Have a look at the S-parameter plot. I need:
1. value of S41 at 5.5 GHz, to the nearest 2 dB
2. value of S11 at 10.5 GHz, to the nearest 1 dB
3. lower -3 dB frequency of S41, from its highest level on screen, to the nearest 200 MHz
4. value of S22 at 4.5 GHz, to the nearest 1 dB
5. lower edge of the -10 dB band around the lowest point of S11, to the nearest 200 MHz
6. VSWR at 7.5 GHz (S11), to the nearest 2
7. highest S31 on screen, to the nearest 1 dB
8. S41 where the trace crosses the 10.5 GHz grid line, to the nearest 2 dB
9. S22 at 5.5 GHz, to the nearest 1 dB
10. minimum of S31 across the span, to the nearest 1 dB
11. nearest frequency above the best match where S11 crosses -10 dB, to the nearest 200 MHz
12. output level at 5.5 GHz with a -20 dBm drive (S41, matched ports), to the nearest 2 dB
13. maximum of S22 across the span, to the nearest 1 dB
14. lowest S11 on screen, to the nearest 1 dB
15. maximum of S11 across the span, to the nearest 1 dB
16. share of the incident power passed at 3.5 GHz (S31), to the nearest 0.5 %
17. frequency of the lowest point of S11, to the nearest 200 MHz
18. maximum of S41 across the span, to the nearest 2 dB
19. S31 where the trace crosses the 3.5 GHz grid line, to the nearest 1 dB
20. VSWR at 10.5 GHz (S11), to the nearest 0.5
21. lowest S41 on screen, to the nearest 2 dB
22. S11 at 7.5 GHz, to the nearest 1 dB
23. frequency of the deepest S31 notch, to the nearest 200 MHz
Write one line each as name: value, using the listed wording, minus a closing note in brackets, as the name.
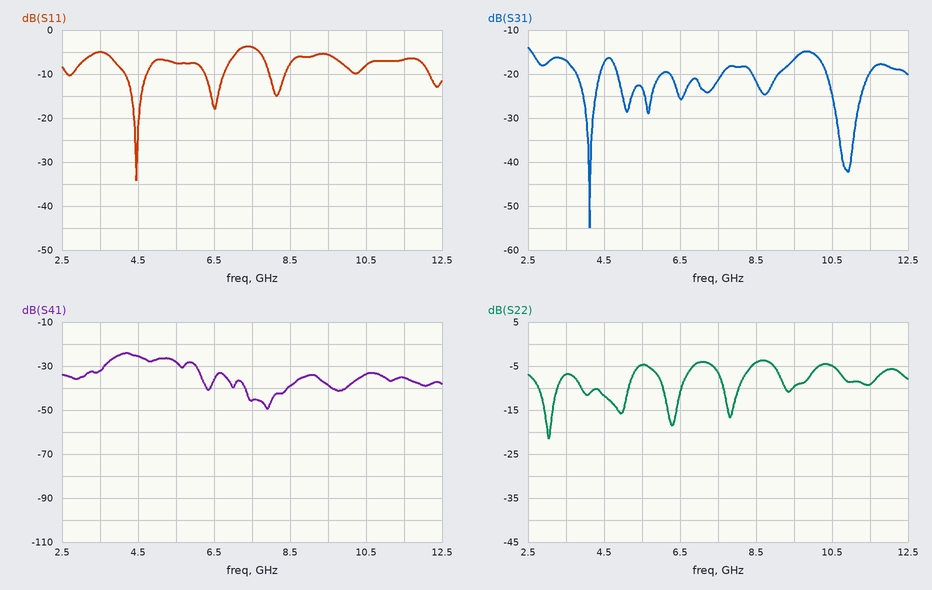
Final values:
value of S41 at 5.5 GHz, to the nearest 2 dB: -28 dB
value of S11 at 10.5 GHz, to the nearest 1 dB: -8 dB
lower -3 dB frequency of S41, from its highest level on screen, to the nearest 200 MHz: 3.8 GHz
value of S22 at 4.5 GHz, to the nearest 1 dB: -12 dB
lower edge of the -10 dB band around the lowest point of S11, to the nearest 200 MHz: 4.2 GHz
VSWR at 7.5 GHz (S11), to the nearest 2: 4
highest S31 on screen, to the nearest 1 dB: -14 dB
S41 where the trace crosses the 10.5 GHz grid line, to the nearest 2 dB: -34 dB
S22 at 5.5 GHz, to the nearest 1 dB: -5 dB
minimum of S31 across the span, to the nearest 1 dB: -55 dB
nearest frequency above the best match where S11 crosses -10 dB, to the nearest 200 MHz: 4.8 GHz
output level at 5.5 GHz with a -20 dBm drive (S41, matched ports), to the nearest 2 dB: -48 dBm
maximum of S22 across the span, to the nearest 1 dB: -4 dB
lowest S11 on screen, to the nearest 1 dB: -34 dB
maximum of S11 across the span, to the nearest 1 dB: -4 dB
share of the incident power passed at 3.5 GHz (S31), to the nearest 0.5 %: 2.0 %
frequency of the lowest point of S11, to the nearest 200 MHz: 4.4 GHz
maximum of S41 across the span, to the nearest 2 dB: -24 dB
S31 where the trace crosses the 3.5 GHz grid line, to the nearest 1 dB: -17 dB
VSWR at 10.5 GHz (S11), to the nearest 0.5: 2.5
lowest S41 on screen, to the nearest 2 dB: -50 dB
S11 at 7.5 GHz, to the nearest 1 dB: -4 dB
frequency of the deepest S31 notch, to the nearest 200 MHz: 4.2 GHz
